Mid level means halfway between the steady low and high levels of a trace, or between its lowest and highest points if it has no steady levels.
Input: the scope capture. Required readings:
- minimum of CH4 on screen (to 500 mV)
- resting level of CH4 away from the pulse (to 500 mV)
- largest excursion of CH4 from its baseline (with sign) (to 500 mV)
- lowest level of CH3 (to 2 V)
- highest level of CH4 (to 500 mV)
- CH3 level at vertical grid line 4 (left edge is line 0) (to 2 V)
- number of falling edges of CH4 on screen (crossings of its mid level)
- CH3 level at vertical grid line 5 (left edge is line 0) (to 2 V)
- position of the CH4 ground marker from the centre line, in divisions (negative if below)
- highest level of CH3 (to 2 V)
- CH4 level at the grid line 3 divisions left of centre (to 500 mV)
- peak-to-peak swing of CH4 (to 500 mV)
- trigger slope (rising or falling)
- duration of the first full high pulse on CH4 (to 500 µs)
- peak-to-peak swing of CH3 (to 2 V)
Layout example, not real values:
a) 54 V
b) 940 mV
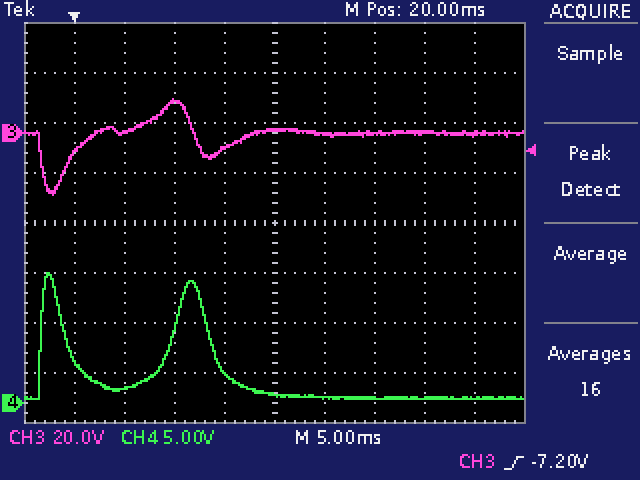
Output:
a) 500 mV
b) 500 mV
c) +12.5 V
d) -24 V
e) 13.0 V
f) -6 V
g) 2
h) 2 V
i) -3.6 div
j) 14 V
k) 1.5 V
l) 12.5 V
m) rising
n) 2.5 ms
o) 38 V
